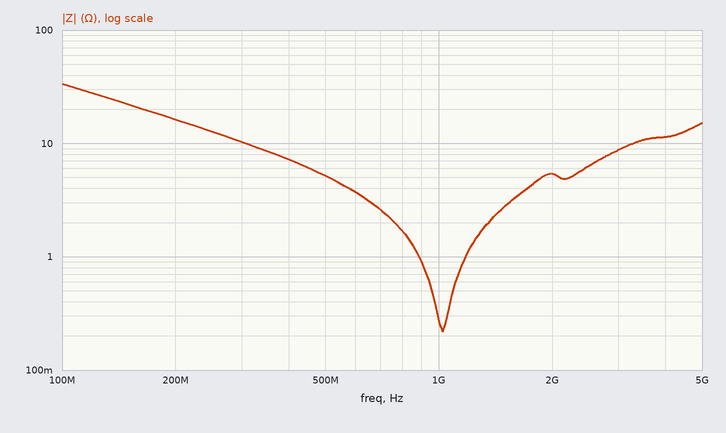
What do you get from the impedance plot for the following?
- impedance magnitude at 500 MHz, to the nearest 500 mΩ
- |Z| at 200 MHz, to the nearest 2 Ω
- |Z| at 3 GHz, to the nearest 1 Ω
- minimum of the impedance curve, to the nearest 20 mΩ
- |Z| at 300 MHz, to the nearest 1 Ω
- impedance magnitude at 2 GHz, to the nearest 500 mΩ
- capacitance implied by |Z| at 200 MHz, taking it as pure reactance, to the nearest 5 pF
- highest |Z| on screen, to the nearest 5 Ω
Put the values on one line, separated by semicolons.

5.0 Ω; 16 Ω; 9 Ω; 220 mΩ; 10 Ω; 5.5 Ω; 50 pF; 35 Ω
